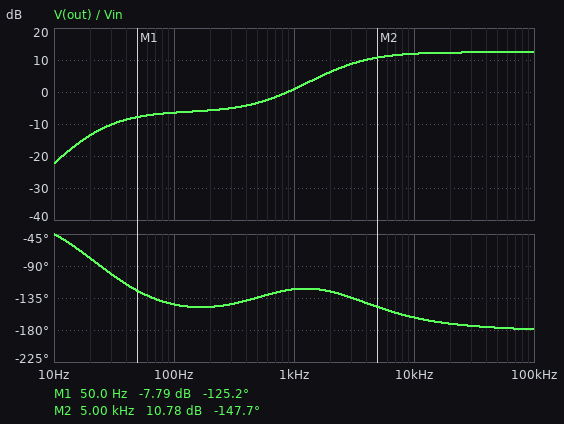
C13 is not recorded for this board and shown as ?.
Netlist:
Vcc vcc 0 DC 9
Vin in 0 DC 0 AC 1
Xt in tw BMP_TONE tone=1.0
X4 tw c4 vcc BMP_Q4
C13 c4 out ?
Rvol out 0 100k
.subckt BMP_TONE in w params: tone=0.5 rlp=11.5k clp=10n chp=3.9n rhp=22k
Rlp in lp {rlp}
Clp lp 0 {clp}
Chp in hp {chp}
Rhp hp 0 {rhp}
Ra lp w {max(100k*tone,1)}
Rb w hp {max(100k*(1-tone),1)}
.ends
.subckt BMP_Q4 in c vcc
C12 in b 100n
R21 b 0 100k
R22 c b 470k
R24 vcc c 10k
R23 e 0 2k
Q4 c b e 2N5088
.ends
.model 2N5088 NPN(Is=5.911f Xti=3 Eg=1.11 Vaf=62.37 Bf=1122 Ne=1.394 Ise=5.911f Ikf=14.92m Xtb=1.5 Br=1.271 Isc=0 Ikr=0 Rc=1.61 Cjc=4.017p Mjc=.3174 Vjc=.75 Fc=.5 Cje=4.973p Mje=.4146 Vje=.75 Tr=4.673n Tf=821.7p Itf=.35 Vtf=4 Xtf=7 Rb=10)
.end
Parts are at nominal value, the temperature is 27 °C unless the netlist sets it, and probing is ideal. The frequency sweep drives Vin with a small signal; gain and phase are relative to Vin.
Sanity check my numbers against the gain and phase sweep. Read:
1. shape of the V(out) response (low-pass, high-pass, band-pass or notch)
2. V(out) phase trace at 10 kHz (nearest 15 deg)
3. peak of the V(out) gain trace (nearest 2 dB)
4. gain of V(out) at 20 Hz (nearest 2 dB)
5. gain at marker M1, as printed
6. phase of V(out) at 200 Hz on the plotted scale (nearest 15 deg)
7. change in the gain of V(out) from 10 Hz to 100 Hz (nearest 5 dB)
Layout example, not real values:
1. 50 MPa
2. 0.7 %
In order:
1. high-pass
2. -165 deg
3. 12 dB
4. -14 dB
5. -7.79 dB
6. -150 deg
7. 15 dB
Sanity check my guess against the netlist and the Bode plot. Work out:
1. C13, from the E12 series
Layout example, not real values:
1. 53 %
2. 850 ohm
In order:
1. 68 nF
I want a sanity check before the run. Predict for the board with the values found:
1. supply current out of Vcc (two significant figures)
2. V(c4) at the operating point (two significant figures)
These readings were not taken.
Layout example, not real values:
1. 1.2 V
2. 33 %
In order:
1. 250 µA
2. 6.5 V
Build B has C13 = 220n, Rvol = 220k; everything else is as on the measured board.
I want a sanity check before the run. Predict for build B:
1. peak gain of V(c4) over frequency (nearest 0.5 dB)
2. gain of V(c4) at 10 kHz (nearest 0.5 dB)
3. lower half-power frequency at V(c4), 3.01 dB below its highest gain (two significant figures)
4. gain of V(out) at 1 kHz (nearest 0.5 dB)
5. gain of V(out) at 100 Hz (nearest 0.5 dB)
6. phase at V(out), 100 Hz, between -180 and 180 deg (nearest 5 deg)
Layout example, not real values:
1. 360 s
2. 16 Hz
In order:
1. 13.0 dB
2. 12.5 dB
3. 3.5 kHz
4. 1.5 dB
5. -6.0 dB
6. -155 deg
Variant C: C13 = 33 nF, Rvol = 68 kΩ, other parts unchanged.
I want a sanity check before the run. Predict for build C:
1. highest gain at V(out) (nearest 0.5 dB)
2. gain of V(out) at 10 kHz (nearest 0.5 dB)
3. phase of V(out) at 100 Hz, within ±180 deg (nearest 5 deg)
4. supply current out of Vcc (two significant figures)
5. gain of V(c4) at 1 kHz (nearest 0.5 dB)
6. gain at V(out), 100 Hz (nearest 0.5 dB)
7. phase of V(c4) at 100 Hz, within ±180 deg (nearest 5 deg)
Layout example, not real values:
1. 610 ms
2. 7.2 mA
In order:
1. 12.0 dB
2. 11.5 dB
3. -125 deg
4. 250 µA
5. 0.5 dB
6. -8.0 dB
7. -160 deg
